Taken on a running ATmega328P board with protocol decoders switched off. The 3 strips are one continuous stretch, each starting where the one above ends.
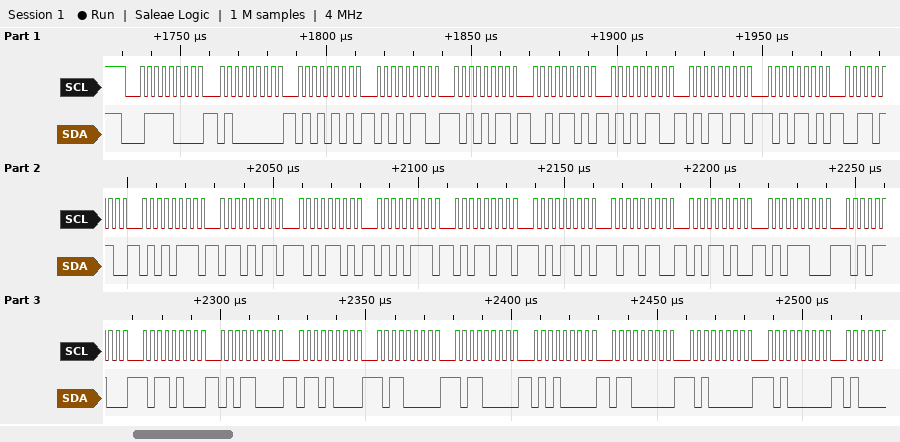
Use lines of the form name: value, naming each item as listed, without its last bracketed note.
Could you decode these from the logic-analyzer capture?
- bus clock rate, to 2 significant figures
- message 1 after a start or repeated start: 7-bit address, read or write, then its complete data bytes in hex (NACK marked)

bus clock rate, to 2 significant figures: 400 kHz
message 1 after a start or repeated start: 7-bit address, read or write, then its complete data bytes in hex: 0x3C write: 40 55 56 AB 2D 56 5B AD 36 57 6B AD 57 5B AD B6 5A 5C AC B4 58 68 B0 B0 50 60 A0 A0
